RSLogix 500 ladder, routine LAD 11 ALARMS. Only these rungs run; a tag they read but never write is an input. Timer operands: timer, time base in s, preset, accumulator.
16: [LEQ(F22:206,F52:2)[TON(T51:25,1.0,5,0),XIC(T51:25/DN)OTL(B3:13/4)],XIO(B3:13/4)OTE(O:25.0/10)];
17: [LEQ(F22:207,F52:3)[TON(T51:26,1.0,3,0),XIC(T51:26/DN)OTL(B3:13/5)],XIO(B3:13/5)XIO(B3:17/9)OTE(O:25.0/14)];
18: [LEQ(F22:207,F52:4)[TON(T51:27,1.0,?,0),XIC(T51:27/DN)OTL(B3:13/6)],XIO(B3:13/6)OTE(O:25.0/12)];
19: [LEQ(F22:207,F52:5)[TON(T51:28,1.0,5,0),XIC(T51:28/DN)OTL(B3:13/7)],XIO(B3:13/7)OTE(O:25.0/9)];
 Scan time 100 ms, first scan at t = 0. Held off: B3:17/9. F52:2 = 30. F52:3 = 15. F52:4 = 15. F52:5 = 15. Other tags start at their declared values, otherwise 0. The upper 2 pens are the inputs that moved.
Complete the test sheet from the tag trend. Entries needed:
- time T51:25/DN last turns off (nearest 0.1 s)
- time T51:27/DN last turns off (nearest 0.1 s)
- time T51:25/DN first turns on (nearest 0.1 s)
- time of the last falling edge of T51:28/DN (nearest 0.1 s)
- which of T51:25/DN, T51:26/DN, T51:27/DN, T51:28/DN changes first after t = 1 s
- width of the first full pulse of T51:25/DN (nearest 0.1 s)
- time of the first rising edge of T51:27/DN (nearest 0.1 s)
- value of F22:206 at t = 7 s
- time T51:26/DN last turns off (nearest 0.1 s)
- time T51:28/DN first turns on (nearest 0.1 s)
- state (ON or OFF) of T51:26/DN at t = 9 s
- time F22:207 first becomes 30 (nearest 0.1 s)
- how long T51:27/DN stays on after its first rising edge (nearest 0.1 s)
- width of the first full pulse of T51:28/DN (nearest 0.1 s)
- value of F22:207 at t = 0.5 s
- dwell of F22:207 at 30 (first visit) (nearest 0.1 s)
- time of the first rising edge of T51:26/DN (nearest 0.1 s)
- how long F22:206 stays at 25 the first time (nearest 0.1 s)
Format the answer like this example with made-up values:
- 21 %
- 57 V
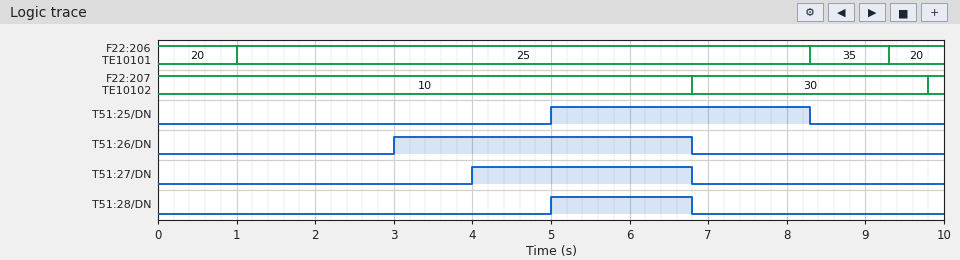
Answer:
- 8.3 s
- 6.8 s
- 5.0 s
- 6.8 s
- T51:26/DN
- 3.3 s
- 4.0 s
- 25
- 6.8 s
- 5.0 s
- OFF
- 6.8 s
- 2.8 s
- 1.8 s
- 10
- 3.0 s
- 3.0 s
- 7.3 s
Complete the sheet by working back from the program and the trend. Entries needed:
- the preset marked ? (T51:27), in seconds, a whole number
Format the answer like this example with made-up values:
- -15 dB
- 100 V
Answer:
- 4 s
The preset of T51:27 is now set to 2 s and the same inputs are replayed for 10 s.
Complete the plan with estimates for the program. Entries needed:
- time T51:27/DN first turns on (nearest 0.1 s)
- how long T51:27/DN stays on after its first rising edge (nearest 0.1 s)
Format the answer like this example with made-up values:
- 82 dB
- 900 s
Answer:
- 2.0 s
- 4.8 s
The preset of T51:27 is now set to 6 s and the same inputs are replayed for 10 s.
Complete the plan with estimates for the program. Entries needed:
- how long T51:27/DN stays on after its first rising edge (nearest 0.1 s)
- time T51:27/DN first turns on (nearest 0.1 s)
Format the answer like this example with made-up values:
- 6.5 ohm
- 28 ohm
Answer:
- 0.8 s
- 6.0 s
